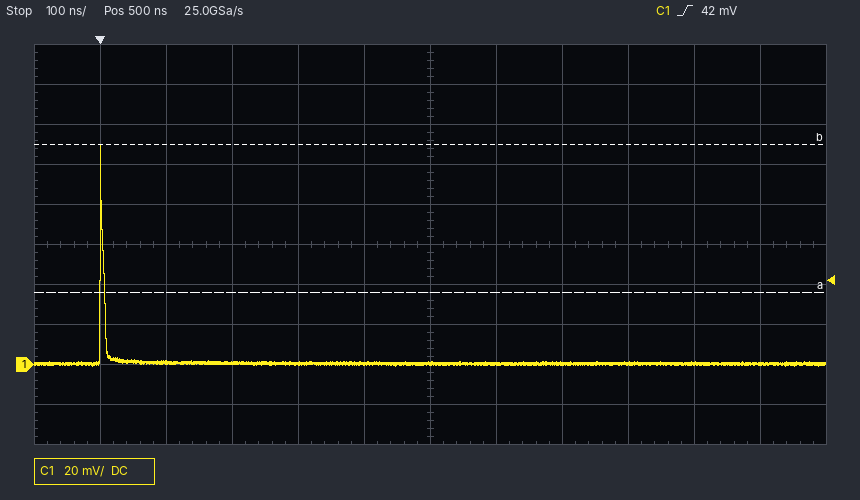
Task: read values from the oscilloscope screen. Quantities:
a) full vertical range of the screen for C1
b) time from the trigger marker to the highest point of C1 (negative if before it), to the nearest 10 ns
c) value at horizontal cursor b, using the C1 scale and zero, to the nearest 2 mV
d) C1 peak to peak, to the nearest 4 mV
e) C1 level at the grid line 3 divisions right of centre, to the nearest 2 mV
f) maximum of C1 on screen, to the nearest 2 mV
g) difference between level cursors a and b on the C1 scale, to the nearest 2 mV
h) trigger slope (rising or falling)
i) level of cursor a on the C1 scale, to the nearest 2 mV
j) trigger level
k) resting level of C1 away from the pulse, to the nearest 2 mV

200 mV
0 ns
110 mV
112 mV
0 mV
110 mV
74 mV
rising
36 mV
42 mV
0 mV
